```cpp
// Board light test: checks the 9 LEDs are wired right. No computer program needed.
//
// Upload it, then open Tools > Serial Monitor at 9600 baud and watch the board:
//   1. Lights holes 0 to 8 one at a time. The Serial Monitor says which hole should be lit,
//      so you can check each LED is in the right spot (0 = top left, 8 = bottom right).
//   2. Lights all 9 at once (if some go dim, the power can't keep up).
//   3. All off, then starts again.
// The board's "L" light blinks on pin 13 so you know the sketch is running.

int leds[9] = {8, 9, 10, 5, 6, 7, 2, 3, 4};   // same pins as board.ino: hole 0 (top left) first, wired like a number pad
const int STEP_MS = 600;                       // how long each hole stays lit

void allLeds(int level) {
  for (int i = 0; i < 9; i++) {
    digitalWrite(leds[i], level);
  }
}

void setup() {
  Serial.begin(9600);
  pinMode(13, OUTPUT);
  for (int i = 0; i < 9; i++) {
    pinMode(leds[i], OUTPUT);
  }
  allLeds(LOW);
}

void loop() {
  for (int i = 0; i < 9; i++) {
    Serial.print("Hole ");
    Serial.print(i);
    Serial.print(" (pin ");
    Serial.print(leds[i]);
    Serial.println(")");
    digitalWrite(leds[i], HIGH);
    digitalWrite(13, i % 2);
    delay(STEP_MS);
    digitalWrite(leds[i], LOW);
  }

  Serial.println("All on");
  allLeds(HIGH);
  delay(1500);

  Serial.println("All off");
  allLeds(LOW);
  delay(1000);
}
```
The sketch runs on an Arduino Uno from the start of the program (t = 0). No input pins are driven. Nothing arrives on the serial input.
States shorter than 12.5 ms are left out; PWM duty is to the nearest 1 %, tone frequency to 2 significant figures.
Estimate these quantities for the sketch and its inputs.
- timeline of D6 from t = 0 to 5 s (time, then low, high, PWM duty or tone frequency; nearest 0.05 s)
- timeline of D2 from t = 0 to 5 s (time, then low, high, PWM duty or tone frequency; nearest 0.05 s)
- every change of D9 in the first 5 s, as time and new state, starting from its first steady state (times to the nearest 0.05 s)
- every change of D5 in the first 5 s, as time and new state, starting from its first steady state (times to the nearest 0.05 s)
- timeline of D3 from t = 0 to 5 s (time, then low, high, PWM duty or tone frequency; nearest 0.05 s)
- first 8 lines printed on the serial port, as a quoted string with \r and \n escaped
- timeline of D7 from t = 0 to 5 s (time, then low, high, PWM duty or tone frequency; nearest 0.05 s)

0 s low; 2.4 s high; 3 s low
0 s low; 3.6 s high; 4.2 s low
0 s low; 0.6 s high; 1.2 s low
0 s low; 1.8 s high; 2.4 s low
0 s low; 4.2 s high; 4.8 s low
"Hole 0 (pin 8)\r\nHole 1 (pin 9)\r\nHole 2 (pin 10)\r\nHole 3 (pin 5)\r\nHole 4 (pin 6)\r\nHole 5 (pin 7)\r\nHole 6 (pin 2)\r\nHole 7 (pin 3)\r\n"
0 s low; 3 s high; 3.6 s low
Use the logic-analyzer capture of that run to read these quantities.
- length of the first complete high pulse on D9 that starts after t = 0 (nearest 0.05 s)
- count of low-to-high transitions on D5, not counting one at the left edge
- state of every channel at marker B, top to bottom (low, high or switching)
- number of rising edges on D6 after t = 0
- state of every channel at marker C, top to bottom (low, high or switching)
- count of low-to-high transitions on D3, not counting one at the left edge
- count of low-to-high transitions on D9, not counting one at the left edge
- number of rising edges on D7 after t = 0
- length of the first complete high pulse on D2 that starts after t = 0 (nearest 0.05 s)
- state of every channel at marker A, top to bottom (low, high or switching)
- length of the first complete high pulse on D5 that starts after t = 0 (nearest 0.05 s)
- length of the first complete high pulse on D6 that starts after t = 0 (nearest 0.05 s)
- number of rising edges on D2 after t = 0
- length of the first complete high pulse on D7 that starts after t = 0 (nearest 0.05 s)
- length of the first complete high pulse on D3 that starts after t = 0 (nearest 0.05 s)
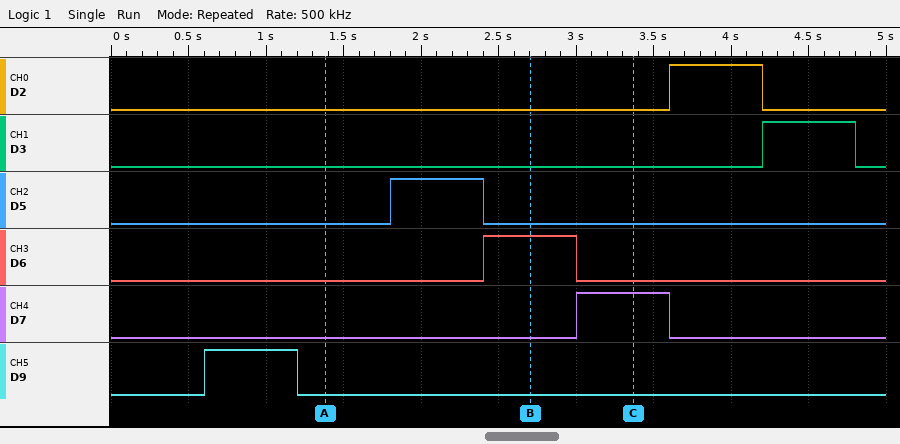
0.60 s
1
D2 low, D3 low, D5 low, D6 high, D7 low, D9 low
1
D2 low, D3 low, D5 low, D6 low, D7 high, D9 low
1
1
1
0.60 s
D2 low, D3 low, D5 low, D6 low, D7 low, D9 low
0.60 s
0.60 s
1
0.60 s
0.60 s
